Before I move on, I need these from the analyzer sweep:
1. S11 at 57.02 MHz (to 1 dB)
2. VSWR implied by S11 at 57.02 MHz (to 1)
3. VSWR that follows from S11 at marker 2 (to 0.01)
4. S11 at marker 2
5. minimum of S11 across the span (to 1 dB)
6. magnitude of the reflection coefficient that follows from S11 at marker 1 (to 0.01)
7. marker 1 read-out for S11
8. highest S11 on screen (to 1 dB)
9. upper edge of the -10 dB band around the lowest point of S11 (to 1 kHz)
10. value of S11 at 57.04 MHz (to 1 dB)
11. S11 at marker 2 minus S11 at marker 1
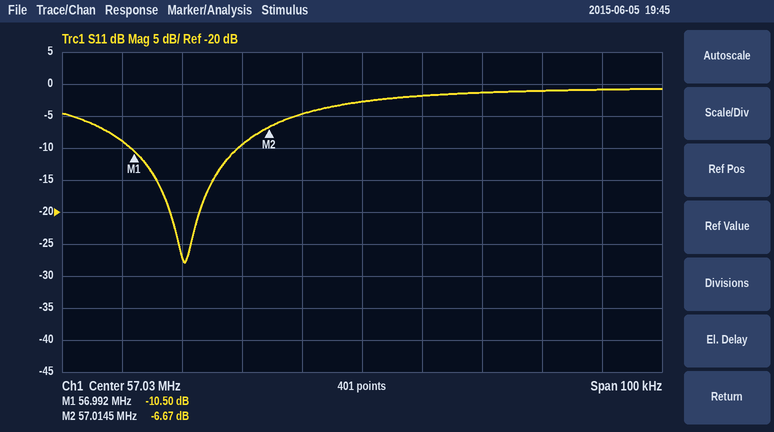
-5 dB
4
2.73
-6.67 dB
-28 dB
0.30
-10.50 dB
-1 dB
57.009 MHz
-2 dB
3.83 dB
